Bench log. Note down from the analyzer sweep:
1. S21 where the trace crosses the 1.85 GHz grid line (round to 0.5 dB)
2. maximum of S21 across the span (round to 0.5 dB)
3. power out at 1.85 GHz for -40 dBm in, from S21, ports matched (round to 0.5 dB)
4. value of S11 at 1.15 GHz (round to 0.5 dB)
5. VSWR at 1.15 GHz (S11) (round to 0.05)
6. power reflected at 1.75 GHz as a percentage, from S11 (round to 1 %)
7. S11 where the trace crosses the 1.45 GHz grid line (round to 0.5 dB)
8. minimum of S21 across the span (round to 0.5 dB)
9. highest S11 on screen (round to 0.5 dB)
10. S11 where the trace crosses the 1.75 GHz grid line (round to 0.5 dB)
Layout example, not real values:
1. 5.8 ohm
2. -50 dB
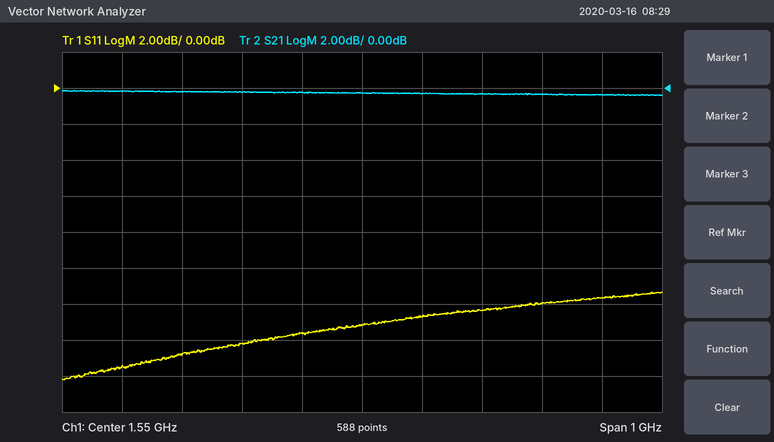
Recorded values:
1. -0.5 dB
2. 0.0 dB
3. -40.5 dBm
4. -15.5 dB
5. 1.40
6. 6 %
7. -13.5 dB
8. -0.5 dB
9. -11.5 dB
10. -12.5 dB
